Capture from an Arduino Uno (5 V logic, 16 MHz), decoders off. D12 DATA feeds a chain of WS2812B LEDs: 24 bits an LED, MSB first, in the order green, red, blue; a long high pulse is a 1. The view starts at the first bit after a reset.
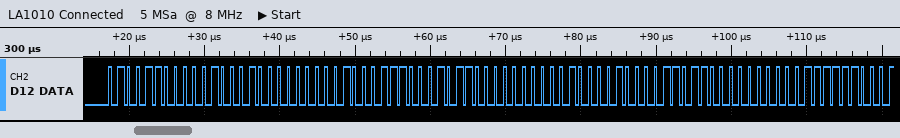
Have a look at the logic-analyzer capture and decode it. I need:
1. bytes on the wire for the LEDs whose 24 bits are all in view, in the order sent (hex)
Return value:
4C 11 00 47 16 00 42 1B 00
